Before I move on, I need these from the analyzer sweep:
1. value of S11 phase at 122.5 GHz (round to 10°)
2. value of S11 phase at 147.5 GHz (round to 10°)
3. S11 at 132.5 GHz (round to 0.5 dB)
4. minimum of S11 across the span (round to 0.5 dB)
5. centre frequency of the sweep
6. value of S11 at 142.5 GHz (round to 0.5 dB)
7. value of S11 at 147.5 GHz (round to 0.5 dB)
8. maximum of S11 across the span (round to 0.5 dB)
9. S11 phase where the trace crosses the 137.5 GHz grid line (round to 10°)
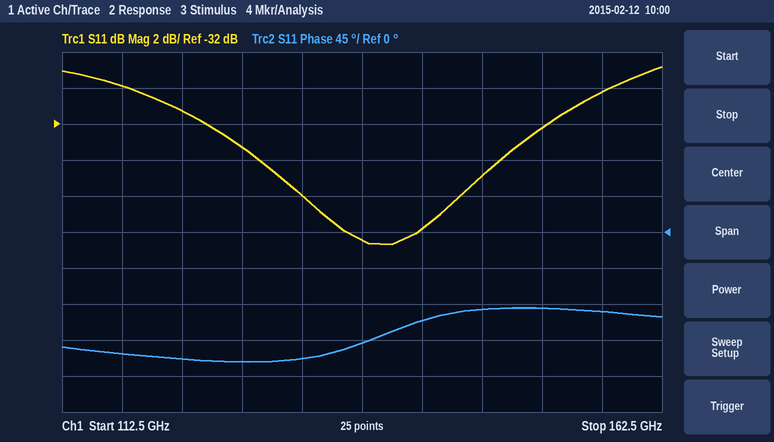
-160°
-100°
-36.0 dB
-38.5 dB
137.5 GHz
-38.0 dB
-35.0 dB
-29.0 dB
-140°
